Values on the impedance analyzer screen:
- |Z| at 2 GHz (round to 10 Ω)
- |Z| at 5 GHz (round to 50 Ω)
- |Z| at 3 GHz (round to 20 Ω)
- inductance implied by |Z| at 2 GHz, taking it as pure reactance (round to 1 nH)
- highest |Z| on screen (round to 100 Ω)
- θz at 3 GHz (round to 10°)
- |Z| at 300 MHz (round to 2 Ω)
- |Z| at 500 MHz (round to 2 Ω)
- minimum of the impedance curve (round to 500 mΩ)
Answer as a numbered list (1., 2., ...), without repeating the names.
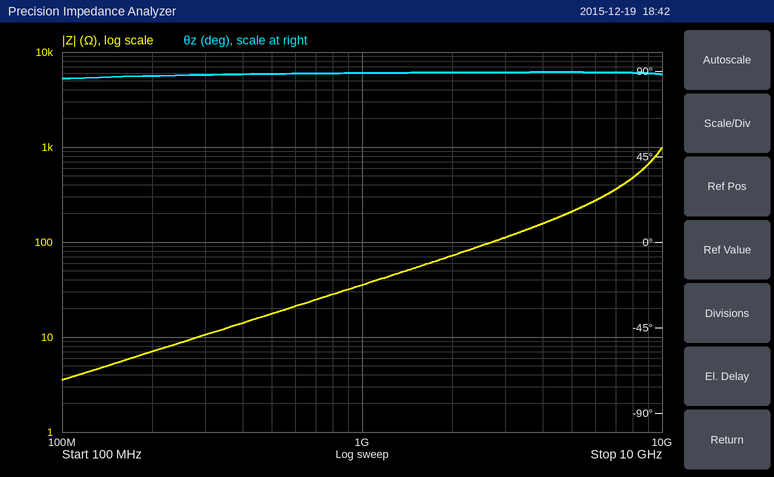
1. 70 Ω
2. 200 Ω
3. 120 Ω
4. 6 nH
5. 1.0 kΩ
6. 90°
7. 10 Ω
8. 18 Ω
9. 3.5 Ω
